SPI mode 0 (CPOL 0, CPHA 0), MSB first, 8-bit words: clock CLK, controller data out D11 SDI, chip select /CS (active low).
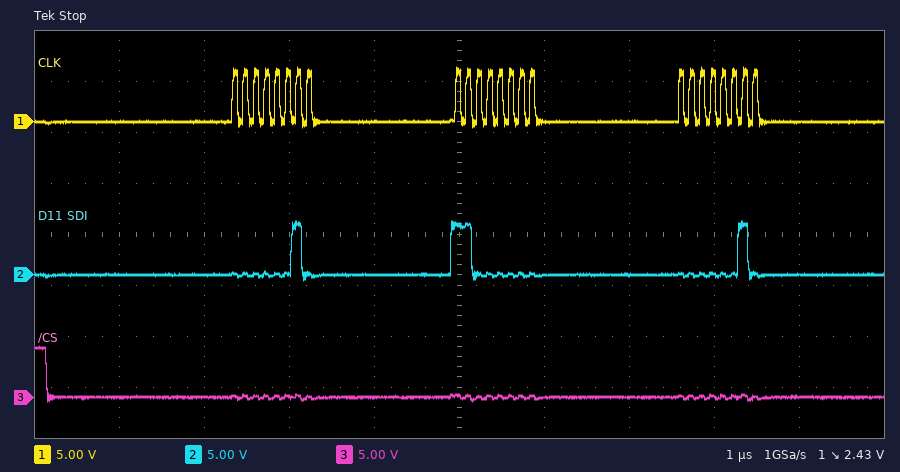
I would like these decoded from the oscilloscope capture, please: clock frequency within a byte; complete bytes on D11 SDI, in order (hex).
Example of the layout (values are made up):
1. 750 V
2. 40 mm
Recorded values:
1. 8 MHz
2. 02 C0 02
